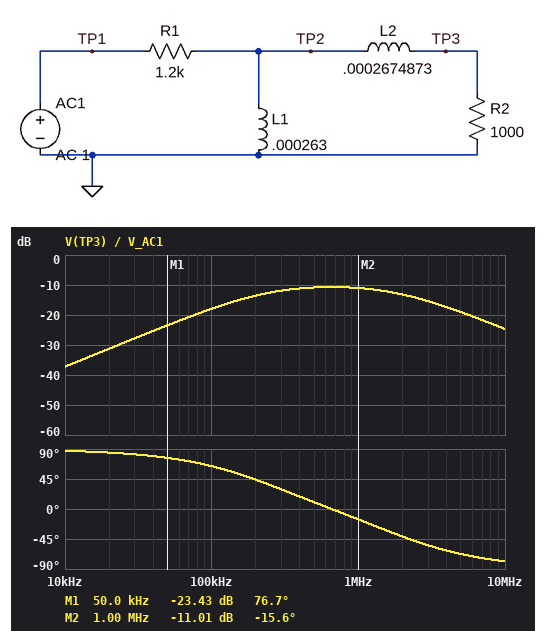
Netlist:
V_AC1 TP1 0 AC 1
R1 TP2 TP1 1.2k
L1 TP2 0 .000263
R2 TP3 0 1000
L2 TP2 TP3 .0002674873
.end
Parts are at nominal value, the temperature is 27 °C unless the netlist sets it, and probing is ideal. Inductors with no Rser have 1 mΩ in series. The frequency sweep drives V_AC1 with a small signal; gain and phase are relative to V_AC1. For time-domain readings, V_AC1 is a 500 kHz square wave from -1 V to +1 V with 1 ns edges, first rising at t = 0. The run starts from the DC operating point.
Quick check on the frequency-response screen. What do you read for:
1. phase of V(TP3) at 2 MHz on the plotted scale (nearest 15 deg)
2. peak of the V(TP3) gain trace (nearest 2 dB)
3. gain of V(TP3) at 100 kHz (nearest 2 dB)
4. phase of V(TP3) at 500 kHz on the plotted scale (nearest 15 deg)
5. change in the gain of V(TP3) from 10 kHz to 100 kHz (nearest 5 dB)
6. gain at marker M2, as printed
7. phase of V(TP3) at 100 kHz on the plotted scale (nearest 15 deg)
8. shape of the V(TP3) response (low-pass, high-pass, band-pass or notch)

-45 deg
-10 dB
-18 dB
15 deg
20 dB
-11.01 dB
60 deg
band-pass
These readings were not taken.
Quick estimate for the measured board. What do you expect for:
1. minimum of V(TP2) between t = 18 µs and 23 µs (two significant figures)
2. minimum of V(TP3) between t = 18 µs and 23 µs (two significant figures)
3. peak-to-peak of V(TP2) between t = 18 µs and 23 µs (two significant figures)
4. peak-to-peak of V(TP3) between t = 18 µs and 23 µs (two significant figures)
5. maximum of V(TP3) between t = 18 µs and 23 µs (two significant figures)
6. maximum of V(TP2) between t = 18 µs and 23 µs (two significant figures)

-1.9 V
-390 mV
3.8 V
770 mV
390 mV
1.9 V
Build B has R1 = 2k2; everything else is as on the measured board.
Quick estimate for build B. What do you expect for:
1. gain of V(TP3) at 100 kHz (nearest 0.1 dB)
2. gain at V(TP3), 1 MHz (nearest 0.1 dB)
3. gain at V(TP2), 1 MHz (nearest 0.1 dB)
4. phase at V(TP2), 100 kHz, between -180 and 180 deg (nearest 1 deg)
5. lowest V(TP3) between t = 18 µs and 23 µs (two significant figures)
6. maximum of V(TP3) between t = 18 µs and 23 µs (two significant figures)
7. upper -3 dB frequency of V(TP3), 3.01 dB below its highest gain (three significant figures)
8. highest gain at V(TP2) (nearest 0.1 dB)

-23.1 dB
-14.7 dB
-8.9 dB
77 deg
-260 mV
260 mV
3.46 MHz
0 dB
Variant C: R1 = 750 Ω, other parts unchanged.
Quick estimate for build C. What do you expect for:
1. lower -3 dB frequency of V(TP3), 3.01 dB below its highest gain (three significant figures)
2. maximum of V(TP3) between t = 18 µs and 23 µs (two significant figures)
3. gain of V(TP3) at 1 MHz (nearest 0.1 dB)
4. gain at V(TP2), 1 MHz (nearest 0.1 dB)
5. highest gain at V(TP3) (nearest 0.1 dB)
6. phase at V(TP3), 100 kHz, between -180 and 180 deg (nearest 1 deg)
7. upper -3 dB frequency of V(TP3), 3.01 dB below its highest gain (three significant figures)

163 kHz
490 mV
-8.9 dB
-3.1 dB
-8.0 dB
60 deg
1.66 MHz
